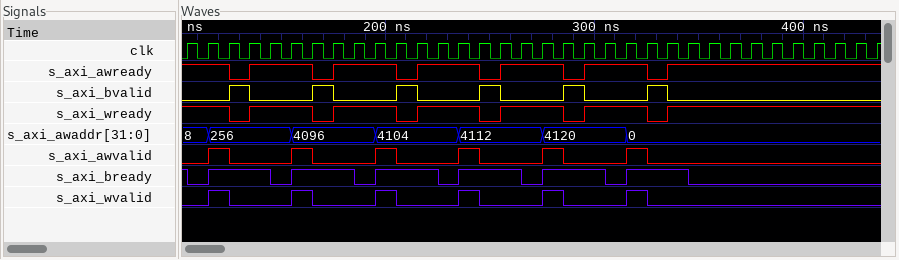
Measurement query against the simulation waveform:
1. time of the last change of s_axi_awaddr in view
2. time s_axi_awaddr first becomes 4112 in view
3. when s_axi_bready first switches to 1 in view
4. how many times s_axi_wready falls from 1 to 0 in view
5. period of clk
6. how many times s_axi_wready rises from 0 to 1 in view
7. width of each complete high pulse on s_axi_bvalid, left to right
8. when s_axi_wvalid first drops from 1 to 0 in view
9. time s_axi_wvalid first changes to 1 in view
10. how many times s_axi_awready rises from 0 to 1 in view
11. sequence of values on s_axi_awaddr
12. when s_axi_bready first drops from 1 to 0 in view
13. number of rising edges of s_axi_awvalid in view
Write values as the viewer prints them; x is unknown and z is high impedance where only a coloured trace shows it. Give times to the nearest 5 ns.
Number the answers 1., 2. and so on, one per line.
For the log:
1. 315 ns
2. 235 ns
3. 115 ns
4. 6
5. 10 ns
6. 6
7. 10 ns, 10 ns, 10 ns, 10 ns, 10 ns, 10 ns
8. 125 ns
9. 115 ns
10. 6
11. 8, 256, 4096, 4104, 4112, 4120, 0
12. 105 ns
13. 6
